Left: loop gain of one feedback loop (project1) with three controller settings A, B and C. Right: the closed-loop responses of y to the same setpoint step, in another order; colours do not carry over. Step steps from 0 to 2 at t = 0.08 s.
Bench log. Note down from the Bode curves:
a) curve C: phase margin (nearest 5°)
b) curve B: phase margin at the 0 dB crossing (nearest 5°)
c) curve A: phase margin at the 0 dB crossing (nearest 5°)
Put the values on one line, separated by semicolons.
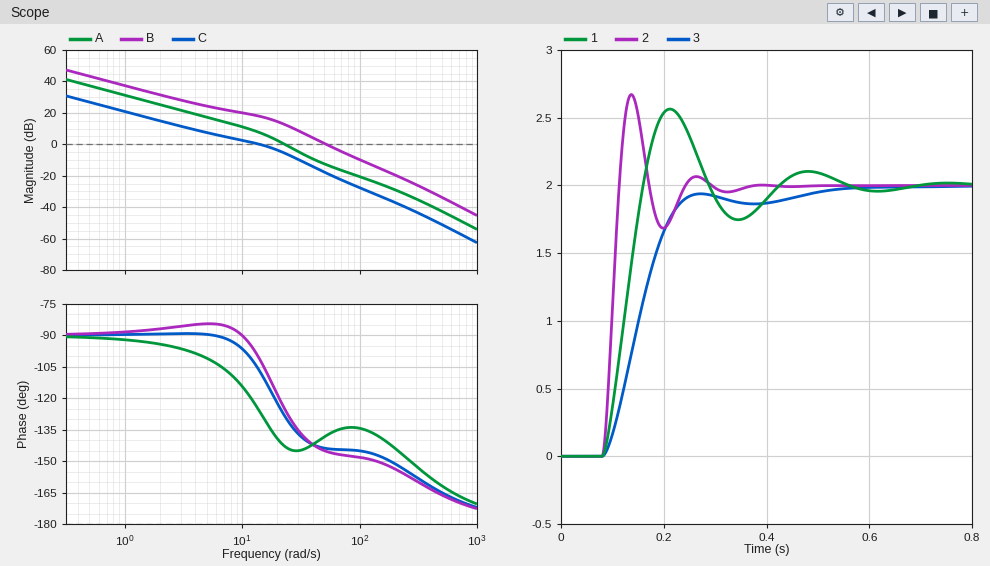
75°; 35°; 35°
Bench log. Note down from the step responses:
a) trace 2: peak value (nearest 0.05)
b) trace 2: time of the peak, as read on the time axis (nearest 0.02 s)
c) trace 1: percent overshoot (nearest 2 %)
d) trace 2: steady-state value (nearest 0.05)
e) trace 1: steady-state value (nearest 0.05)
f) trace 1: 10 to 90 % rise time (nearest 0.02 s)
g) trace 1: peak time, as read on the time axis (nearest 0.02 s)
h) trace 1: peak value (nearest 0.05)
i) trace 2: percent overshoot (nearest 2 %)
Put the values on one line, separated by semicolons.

2.65; 0.14 s; 28 %; 2.00; 2.00; 0.06 s; 0.22 s; 2.55; 34 %
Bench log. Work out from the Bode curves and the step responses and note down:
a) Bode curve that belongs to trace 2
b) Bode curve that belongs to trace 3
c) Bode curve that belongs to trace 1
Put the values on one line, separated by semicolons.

B; C; A
